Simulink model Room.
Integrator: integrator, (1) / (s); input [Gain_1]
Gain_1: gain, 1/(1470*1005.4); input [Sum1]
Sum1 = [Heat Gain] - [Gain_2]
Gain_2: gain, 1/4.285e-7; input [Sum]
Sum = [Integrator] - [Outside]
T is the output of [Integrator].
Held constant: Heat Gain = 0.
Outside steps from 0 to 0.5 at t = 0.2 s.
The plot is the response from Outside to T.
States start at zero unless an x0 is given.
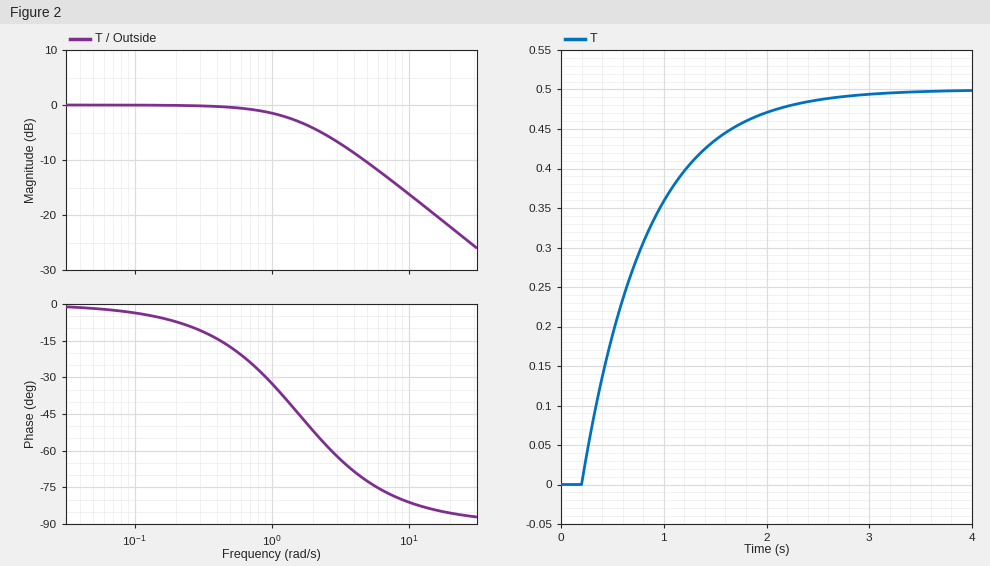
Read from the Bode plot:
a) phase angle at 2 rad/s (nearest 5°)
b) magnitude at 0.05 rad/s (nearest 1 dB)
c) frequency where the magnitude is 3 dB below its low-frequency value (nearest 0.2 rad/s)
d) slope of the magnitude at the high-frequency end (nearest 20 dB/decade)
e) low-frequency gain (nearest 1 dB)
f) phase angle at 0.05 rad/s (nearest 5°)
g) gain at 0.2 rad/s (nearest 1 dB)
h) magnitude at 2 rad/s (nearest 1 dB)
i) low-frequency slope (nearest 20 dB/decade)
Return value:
-50°
0 dB
1.6 rad/s
-20 dB/decade
0 dB
0°
0 dB
-4 dB
0 dB/decade
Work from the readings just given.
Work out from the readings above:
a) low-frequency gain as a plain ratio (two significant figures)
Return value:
1.0
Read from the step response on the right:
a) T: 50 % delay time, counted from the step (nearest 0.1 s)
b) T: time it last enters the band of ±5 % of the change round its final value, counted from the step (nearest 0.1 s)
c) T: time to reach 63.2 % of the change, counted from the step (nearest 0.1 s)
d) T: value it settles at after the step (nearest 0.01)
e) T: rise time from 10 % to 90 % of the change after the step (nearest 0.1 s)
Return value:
0.4 s
1.9 s
0.6 s
0.50
1.4 s
